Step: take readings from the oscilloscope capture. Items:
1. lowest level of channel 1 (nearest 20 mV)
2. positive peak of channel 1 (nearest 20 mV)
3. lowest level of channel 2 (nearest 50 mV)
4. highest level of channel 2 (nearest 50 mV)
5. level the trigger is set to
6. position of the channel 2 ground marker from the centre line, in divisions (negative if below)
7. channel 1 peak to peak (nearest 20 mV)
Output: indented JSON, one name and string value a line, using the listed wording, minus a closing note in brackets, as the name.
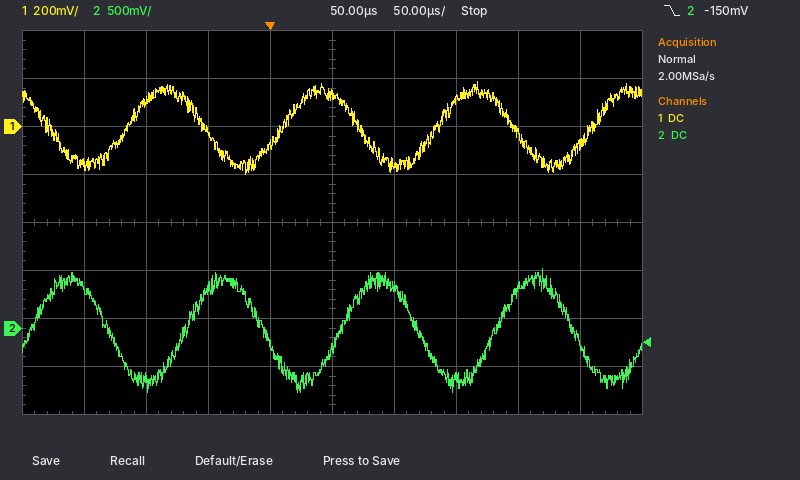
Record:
{
  "lowest level of channel 1": "-200 mV",
  "positive peak of channel 1": "180 mV",
  "lowest level of channel 2": "-650 mV",
  "highest level of channel 2": "600 mV",
  "level the trigger is set to": "-150 mV",
  "position of the channel 2 ground marker from the centre line, in divisions": "-2.2 div",
  "channel 1 peak to peak": "380 mV"
}
